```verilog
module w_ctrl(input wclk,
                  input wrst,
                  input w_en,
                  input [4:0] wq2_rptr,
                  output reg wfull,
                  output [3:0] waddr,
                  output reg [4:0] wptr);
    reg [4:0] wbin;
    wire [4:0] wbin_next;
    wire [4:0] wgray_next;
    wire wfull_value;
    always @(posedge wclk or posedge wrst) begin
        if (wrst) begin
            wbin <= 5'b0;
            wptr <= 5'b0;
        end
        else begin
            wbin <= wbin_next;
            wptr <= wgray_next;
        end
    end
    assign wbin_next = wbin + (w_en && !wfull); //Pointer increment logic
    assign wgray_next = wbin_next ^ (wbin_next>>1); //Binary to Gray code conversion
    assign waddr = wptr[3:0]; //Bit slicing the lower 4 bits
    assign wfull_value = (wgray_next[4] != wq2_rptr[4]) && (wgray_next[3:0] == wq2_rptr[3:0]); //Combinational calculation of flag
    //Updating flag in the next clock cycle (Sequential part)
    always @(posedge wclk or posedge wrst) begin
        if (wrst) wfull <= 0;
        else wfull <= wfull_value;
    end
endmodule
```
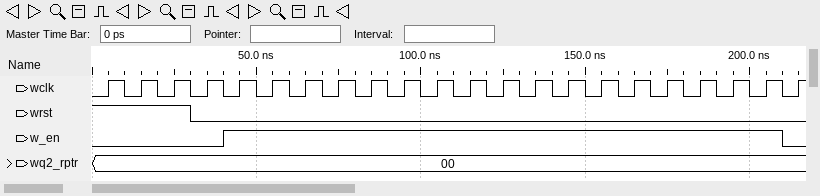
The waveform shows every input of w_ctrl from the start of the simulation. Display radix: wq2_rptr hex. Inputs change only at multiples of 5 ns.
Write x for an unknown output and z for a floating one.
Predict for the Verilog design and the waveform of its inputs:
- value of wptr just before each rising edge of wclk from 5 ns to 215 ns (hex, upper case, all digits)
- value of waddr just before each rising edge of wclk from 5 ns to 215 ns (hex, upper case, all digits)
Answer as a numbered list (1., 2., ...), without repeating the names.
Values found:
1. 00, 00, 00, 00, 00, 01, 03, 02, 06, 07, 05, 04, 0C, 0D, 0F, 0E, 0A, 0B, 09, 08, 18, 19
2. 0, 0, 0, 0, 0, 1, 3, 2, 6, 7, 5, 4, C, D, F, E, A, B, 9, 8, 8, 9
